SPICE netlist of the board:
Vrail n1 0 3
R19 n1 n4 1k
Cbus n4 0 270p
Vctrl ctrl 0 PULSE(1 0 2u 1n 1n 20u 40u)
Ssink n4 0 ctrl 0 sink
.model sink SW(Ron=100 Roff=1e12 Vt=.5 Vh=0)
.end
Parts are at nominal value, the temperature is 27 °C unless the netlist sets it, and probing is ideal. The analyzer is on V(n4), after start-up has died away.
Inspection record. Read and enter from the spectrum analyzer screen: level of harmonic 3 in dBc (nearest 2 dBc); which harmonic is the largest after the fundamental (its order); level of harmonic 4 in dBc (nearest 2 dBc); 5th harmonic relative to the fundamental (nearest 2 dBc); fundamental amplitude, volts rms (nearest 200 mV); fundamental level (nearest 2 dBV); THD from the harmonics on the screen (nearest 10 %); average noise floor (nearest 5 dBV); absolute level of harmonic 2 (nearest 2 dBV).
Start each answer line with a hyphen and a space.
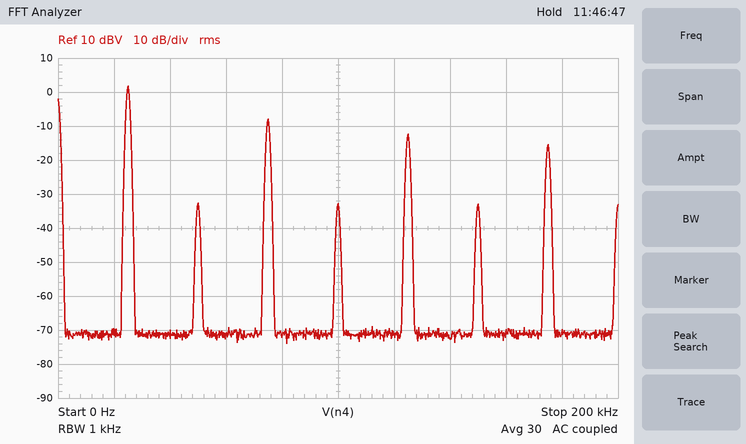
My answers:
- -10 dBc
- 3
- -34 dBc
- -14 dBc
- 1.2 V
- 2 dBV
- 40 %
- -70 dBV
- -32 dBV
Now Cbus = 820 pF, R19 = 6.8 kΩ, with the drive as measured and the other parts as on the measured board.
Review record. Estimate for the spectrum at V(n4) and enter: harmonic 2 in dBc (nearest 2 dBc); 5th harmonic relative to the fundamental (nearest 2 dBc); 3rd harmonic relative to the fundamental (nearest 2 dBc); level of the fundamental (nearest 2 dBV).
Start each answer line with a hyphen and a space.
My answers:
- -12 dBc
- -18 dBc
- -12 dBc
- 0 dBV
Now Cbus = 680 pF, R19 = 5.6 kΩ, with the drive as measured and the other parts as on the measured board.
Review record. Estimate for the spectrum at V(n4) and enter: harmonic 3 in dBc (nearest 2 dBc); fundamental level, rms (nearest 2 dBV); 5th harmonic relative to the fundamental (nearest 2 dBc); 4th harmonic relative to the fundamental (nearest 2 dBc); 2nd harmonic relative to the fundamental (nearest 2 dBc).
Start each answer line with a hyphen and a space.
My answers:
- -12 dBc
- 2 dBV
- -18 dBc
- -18 dBc
- -14 dBc
